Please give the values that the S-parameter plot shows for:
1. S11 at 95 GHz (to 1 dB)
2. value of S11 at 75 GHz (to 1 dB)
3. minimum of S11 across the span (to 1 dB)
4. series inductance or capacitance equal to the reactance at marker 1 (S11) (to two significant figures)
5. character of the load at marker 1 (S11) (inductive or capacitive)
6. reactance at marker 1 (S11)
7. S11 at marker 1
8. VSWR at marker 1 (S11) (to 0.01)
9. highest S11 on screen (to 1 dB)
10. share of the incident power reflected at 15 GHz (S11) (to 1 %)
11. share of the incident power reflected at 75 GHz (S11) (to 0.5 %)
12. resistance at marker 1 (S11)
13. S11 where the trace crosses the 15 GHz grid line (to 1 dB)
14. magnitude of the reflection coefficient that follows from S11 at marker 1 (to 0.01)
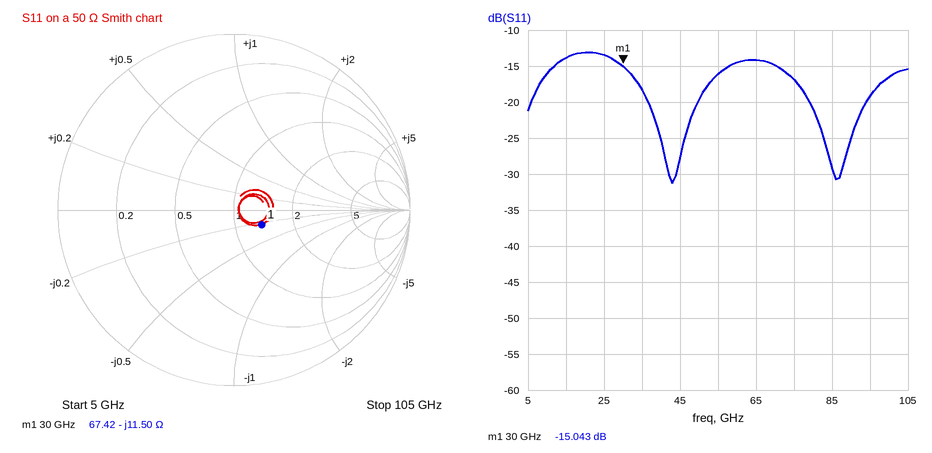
-19 dB
-17 dB
-31 dB
460 fF
capacitive
-11.50 Ω
-15.043 dB
1.43
-13 dB
4 %
2.0 %
67.42 Ω
-14 dB
0.18
